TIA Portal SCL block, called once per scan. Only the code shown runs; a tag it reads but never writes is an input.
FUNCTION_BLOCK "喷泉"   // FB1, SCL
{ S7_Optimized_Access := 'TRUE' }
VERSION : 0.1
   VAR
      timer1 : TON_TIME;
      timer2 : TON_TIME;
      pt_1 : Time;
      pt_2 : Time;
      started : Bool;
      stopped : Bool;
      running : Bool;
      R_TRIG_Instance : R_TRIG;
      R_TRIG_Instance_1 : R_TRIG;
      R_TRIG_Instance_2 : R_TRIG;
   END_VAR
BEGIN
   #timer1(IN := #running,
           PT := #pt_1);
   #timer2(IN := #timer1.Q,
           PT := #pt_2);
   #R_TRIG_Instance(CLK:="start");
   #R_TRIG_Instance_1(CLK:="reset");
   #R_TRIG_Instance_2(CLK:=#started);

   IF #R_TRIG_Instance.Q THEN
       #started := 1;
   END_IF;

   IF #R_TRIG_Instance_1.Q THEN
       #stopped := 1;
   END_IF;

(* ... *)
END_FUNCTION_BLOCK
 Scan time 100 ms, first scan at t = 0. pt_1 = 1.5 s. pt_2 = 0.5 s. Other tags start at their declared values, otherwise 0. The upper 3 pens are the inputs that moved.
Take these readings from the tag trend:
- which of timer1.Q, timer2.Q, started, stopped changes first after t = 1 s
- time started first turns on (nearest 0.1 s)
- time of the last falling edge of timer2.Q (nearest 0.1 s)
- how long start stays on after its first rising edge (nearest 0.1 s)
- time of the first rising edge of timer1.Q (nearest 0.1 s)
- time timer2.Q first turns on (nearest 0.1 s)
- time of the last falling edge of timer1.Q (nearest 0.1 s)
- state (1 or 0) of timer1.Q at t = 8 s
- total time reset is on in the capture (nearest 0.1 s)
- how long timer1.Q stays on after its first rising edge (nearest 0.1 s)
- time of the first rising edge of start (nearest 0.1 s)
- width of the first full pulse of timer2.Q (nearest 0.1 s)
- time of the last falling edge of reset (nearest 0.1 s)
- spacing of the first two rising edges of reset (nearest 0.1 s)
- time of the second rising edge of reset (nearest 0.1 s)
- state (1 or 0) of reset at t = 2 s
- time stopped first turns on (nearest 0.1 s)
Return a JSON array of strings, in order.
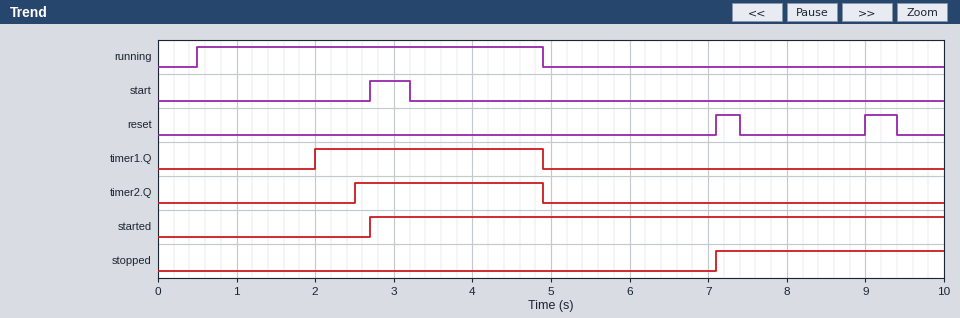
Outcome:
["timer1.Q", "2.7 s", "4.9 s", "0.5 s", "2.0 s", "2.5 s", "4.9 s", "0", "0.7 s", "2.9 s", "2.7 s", "2.4 s", "9.4 s", "1.9 s", "9.0 s", "0", "7.1 s"]
